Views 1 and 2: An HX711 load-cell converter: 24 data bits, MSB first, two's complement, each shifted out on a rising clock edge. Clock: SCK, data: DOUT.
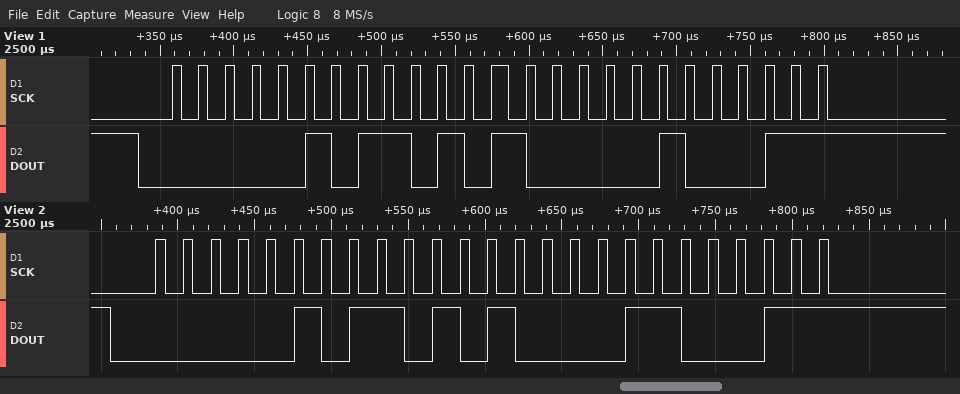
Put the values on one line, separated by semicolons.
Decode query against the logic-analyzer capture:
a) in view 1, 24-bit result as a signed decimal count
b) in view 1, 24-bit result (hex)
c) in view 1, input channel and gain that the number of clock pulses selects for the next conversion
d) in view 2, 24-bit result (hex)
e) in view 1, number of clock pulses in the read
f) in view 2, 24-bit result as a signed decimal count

370723; 0x05A823; channel A, gain 128; 0x05A863; 25; 370787
